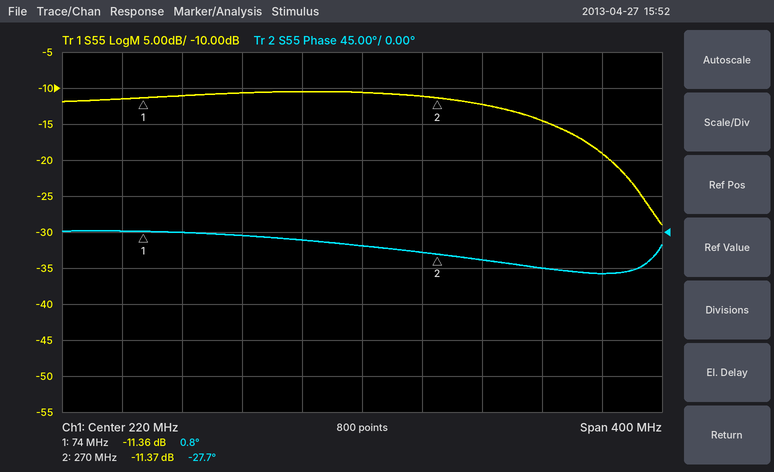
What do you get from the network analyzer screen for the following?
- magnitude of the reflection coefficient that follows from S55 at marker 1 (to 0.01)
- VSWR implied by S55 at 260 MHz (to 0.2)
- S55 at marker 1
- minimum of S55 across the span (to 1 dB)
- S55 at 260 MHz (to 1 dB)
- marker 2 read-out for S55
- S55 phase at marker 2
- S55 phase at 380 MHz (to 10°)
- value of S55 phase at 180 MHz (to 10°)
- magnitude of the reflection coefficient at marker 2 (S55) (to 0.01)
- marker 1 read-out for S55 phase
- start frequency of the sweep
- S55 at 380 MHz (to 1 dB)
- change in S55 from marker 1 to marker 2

0.27
1.8
-11.36 dB
-29 dB
-11 dB
-11.37 dB
-27.7°
-50°
-10°
0.27
0.8°
20 MHz
-19 dB
-0.01 dB
